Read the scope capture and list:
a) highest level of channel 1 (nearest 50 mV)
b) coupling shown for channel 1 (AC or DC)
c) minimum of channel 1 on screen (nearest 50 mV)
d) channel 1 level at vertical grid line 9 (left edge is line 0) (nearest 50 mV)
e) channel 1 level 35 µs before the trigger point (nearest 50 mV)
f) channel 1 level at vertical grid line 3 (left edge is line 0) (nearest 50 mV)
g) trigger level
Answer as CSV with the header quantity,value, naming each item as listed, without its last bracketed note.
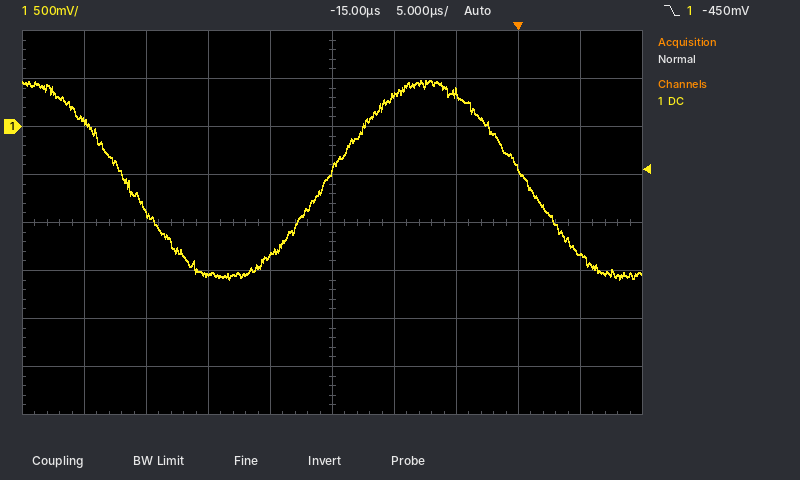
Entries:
quantity,value
highest level of channel 1,500 mV
coupling shown for channel 1,DC
minimum of channel 1 on screen,-1.60 V
channel 1 level at vertical grid line 9 (left edge is line 0),-1.35 V
channel 1 level 35 µs before the trigger point,50 mV
channel 1 level at vertical grid line 3 (left edge is line 0),-1.55 V
trigger level,-450 mV
